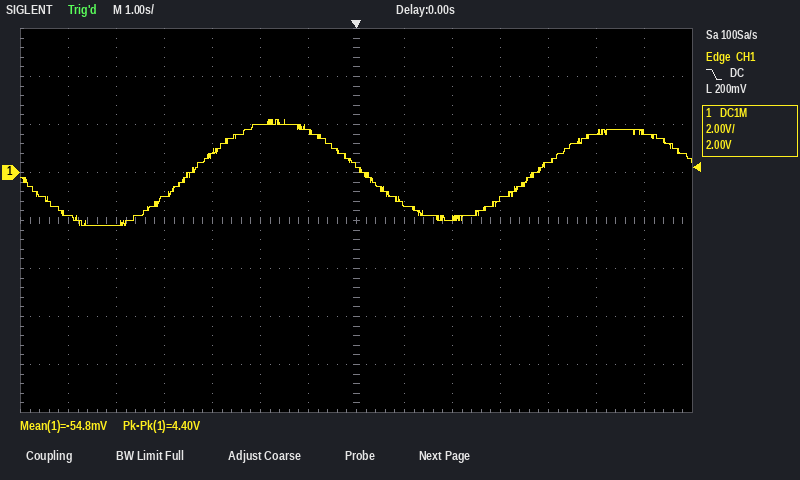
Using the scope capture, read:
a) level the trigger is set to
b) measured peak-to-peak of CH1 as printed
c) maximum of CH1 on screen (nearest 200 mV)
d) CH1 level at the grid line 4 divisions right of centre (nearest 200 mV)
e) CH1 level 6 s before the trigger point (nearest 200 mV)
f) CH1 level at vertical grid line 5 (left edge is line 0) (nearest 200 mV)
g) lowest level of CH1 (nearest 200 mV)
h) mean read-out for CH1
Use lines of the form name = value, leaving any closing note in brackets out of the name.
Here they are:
level the trigger is set to = 200 mV
measured peak-to-peak of CH1 as printed = 4.40 V
maximum of CH1 on screen = 2.2 V
CH1 level at the grid line 4 divisions right of centre = 400 mV
CH1 level 6 s before the trigger point = -1.8 V
CH1 level at vertical grid line 5 (left edge is line 0) = 2.0 V
lowest level of CH1 = -2.2 V
mean read-out for CH1 = -54.8 mV
